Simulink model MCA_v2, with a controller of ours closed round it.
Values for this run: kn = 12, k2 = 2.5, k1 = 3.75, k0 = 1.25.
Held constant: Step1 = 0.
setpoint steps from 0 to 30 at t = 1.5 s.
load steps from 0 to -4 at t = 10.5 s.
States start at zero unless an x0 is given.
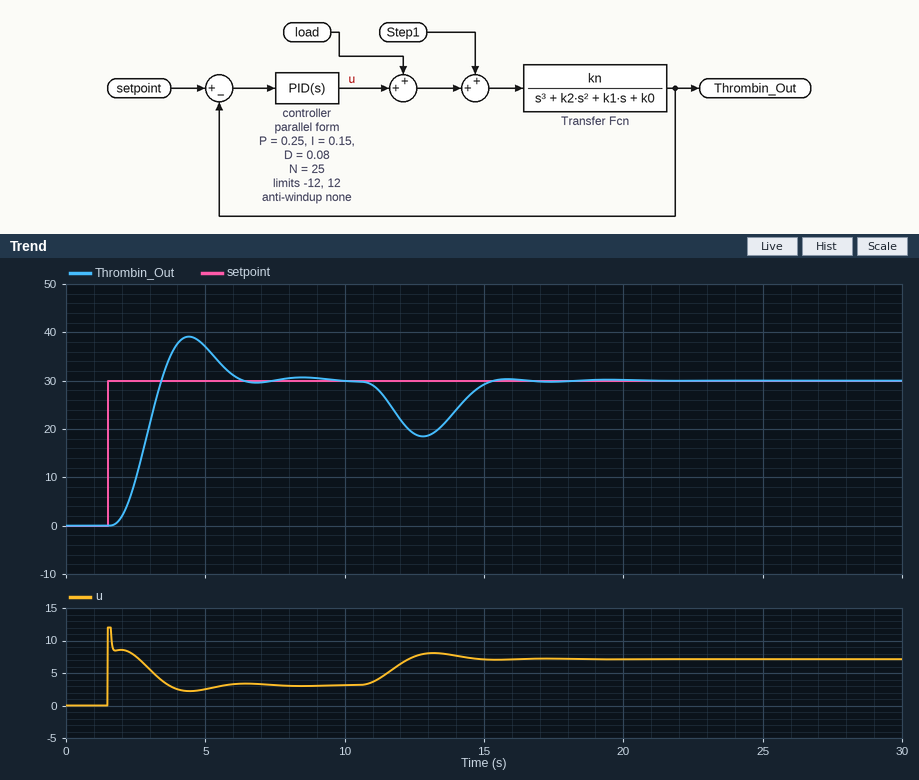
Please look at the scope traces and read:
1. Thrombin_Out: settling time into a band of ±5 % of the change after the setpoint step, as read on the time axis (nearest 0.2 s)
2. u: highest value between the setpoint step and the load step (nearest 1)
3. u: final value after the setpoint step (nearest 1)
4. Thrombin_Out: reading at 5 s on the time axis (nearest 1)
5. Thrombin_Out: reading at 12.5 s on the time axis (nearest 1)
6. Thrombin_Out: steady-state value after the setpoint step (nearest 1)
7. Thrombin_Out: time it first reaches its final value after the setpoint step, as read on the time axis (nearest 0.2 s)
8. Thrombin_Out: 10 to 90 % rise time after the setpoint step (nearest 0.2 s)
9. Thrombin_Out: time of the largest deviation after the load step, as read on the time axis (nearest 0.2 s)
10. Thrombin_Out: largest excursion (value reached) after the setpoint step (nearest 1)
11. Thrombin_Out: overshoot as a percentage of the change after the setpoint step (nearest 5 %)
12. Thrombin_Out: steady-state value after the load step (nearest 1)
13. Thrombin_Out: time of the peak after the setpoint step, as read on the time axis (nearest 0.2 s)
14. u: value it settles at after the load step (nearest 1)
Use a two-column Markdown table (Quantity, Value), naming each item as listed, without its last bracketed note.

| Quantity | Value |
|---|---|
| Thrombin_Out: settling time into a band of ±5 % of the change after the setpoint step, as read on the time axis | 6.0 s |
| u: highest value between the setpoint step and the load step | 12 |
| u: final value after the setpoint step | 3 |
| Thrombin_Out: reading at 5 s on the time axis | 37 |
| Thrombin_Out: reading at 12.5 s on the time axis | 19 |
| Thrombin_Out: steady-state value after the setpoint step | 30 |
| Thrombin_Out: time it first reaches its final value after the setpoint step, as read on the time axis | 3.4 s |
| Thrombin_Out: 10 to 90 % rise time after the setpoint step | 1.2 s |
| Thrombin_Out: time of the largest deviation after the load step, as read on the time axis | 12.8 s |
| Thrombin_Out: largest excursion (value reached) after the setpoint step | 39 |
| Thrombin_Out: overshoot as a percentage of the change after the setpoint step | 30 % |
| Thrombin_Out: steady-state value after the load step | 30 |
| Thrombin_Out: time of the peak after the setpoint step, as read on the time axis | 4.4 s |
| u: value it settles at after the load step | 7 |
